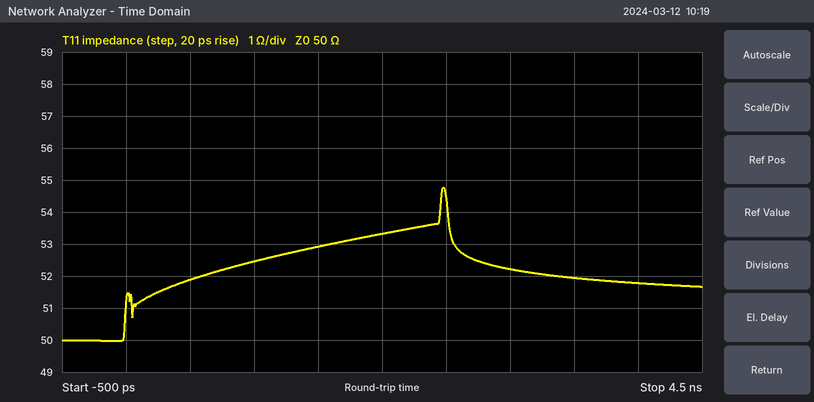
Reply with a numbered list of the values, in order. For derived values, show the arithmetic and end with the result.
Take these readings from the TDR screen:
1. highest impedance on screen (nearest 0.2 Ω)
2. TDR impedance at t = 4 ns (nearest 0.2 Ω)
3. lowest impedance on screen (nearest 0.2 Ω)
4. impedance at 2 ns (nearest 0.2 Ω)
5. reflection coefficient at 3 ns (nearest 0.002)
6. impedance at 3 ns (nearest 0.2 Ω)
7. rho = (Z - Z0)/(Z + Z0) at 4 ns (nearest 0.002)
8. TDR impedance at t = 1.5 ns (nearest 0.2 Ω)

1. 54.8 Ω
2. 51.8 Ω
3. 50.0 Ω
4. 53.4 Ω
5. (52.2 − 50)/(52.2 + 50) ≈ +0.022
6. 52.2 Ω
7. (51.8 − 50)/(51.8 + 50) ≈ +0.018
8. 53.0 Ω
